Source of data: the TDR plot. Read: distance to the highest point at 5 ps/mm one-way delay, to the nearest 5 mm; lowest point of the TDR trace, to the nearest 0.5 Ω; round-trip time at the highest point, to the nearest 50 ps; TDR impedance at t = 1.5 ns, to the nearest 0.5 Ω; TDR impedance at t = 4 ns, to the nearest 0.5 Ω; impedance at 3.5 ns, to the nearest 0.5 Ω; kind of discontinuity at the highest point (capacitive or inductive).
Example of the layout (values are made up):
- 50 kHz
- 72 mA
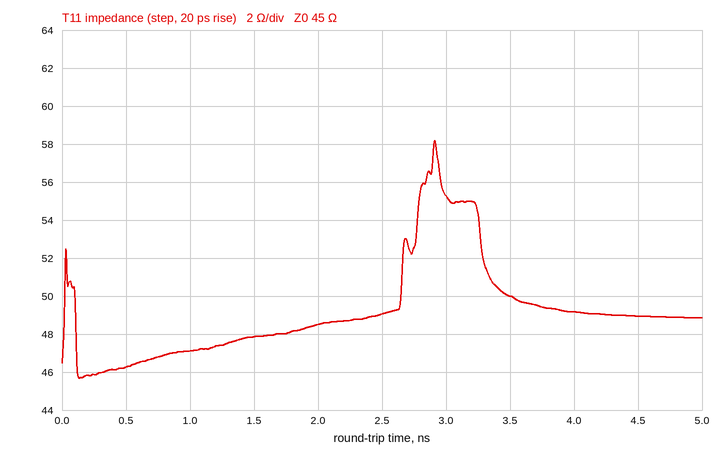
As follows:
- 290 mm
- 45.5 Ω
- 2.90 ns
- 48.0 Ω
- 49.0 Ω
- 50.0 Ω
- inductive
